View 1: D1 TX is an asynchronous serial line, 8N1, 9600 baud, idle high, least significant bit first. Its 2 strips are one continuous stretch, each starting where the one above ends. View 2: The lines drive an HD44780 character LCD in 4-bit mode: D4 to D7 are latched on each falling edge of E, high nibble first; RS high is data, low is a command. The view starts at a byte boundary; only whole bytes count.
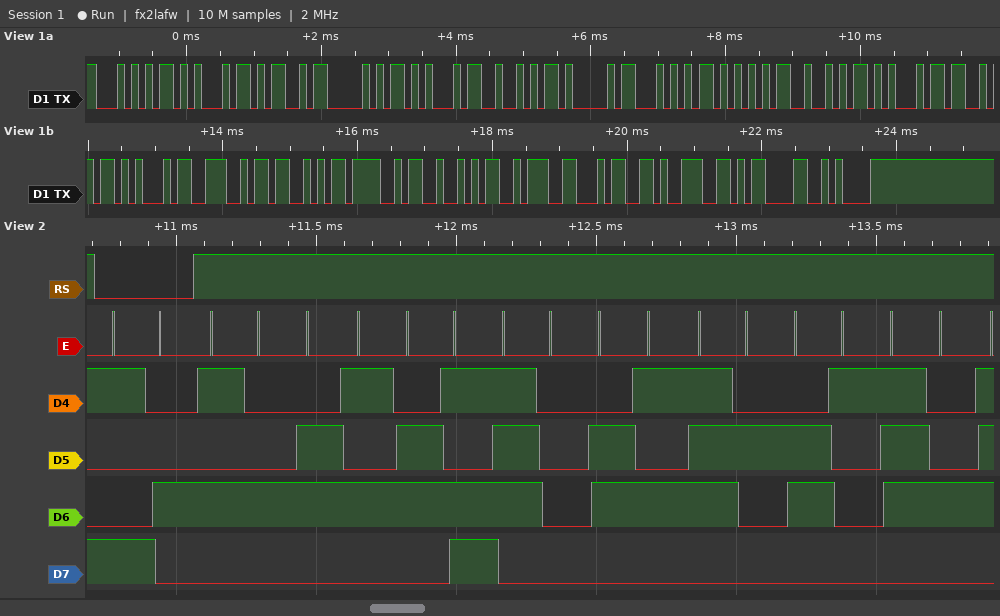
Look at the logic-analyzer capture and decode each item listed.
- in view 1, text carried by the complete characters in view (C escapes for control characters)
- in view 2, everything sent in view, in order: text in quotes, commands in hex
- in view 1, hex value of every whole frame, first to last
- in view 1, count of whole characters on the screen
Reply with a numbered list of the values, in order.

1. "TEMPERATURESENSOR:49\r\n"
2. 0x94 "Temperat"
3. 54 45 4D 50 45 52 41 54 55 52 45 53 45 4E 53 4F 52 3A 34 39 0D 0A
4. 22
